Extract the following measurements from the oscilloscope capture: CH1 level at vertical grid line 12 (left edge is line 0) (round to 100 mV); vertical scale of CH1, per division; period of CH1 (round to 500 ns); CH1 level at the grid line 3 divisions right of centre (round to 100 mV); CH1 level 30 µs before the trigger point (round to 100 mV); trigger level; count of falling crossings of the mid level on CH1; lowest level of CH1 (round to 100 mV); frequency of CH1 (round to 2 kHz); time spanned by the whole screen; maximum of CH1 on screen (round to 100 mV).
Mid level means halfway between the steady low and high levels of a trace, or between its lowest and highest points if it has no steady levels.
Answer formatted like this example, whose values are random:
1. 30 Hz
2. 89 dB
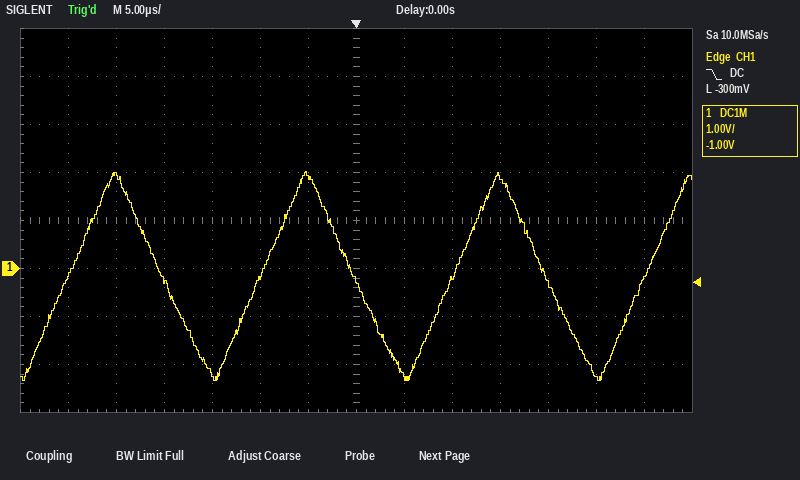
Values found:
1. -2.3 V
2. 1 V
3. 20.0 µs
4. 1.9 V
5. -200 mV
6. -300 mV
7. 3
8. -2.3 V
9. 50 kHz
10. 70 µs
11. 2.0 V
